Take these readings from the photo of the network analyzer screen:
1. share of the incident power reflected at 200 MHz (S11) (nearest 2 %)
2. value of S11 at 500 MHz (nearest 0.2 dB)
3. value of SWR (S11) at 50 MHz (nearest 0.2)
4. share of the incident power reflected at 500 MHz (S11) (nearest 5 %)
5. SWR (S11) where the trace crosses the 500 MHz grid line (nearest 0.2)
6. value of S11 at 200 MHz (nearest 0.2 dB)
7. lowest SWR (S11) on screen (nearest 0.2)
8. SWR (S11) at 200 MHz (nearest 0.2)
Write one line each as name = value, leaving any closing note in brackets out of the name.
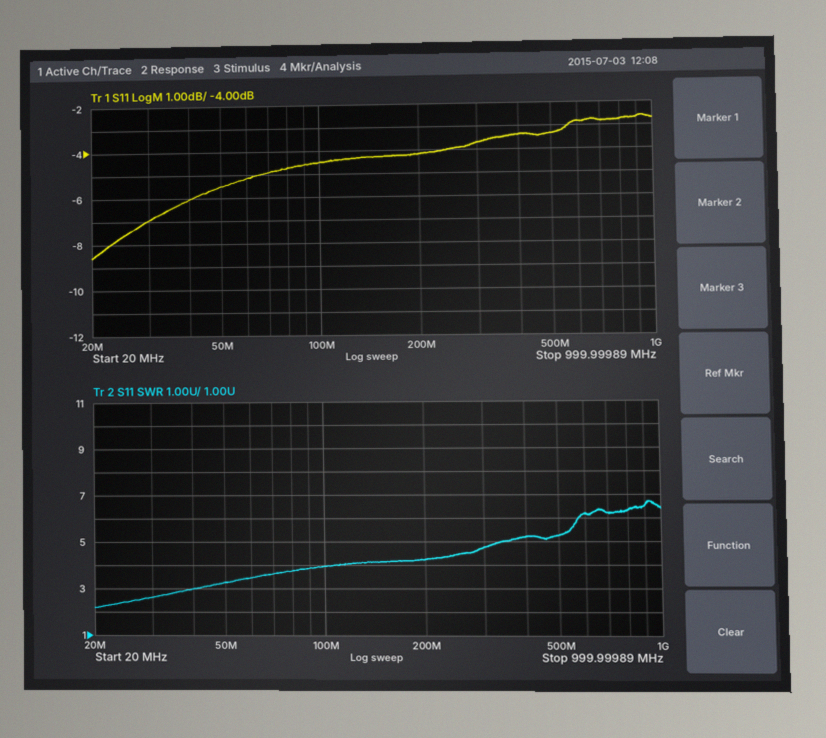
share of the incident power reflected at 200 MHz (S11) = 38 %
value of S11 at 500 MHz = -3.4 dB
value of SWR (S11) at 50 MHz = 3.2
share of the incident power reflected at 500 MHz (S11) = 45 %
SWR (S11) where the trace crosses the 500 MHz grid line = 5.2
value of S11 at 200 MHz = -4.2 dB
lowest SWR (S11) on screen = 2.2
SWR (S11) at 200 MHz = 4.2
